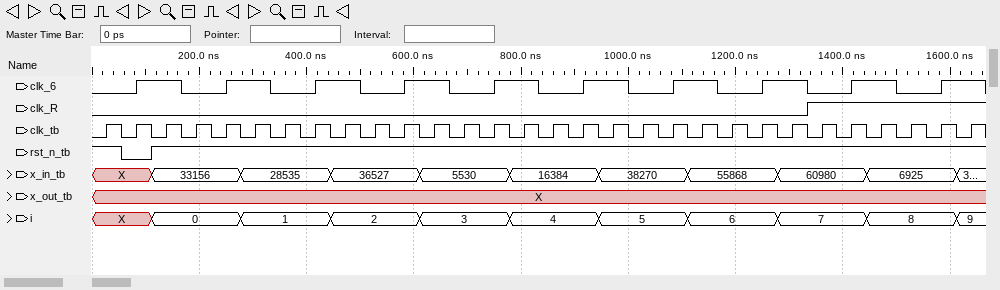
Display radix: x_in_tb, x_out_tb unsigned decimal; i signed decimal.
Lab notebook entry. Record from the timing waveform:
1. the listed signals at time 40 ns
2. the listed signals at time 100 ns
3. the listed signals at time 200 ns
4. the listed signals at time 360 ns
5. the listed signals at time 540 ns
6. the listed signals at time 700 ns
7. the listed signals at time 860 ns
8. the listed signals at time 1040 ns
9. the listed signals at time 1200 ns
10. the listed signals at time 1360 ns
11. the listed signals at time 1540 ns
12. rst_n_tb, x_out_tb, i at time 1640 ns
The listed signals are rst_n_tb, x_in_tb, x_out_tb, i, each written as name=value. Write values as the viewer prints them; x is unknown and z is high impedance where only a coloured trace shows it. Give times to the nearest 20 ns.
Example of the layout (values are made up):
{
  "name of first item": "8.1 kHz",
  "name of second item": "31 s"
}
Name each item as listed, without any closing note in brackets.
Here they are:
{
  "the listed signals at time 40 ns": "rst_n_tb=1, x_in_tb=X, x_out_tb=X, i=X",
  "the listed signals at time 100 ns": "rst_n_tb=0, x_in_tb=X, x_out_tb=X, i=X",
  "the listed signals at time 200 ns": "rst_n_tb=1, x_in_tb=33156, x_out_tb=X, i=0",
  "the listed signals at time 360 ns": "rst_n_tb=1, x_in_tb=28535, x_out_tb=X, i=1",
  "the listed signals at time 540 ns": "rst_n_tb=1, x_in_tb=36527, x_out_tb=X, i=2",
  "the listed signals at time 700 ns": "rst_n_tb=1, x_in_tb=5530, x_out_tb=X, i=3",
  "the listed signals at time 860 ns": "rst_n_tb=1, x_in_tb=16384, x_out_tb=X, i=4",
  "the listed signals at time 1040 ns": "rst_n_tb=1, x_in_tb=38270, x_out_tb=X, i=5",
  "the listed signals at time 1200 ns": "rst_n_tb=1, x_in_tb=55868, x_out_tb=X, i=6",
  "the listed signals at time 1360 ns": "rst_n_tb=1, x_in_tb=60980, x_out_tb=X, i=7",
  "the listed signals at time 1540 ns": "rst_n_tb=1, x_in_tb=6925, x_out_tb=X, i=8",
  "rst_n_tb, x_out_tb, i at time 1640 ns": "rst_n_tb=1, x_out_tb=X, i=9"
}
